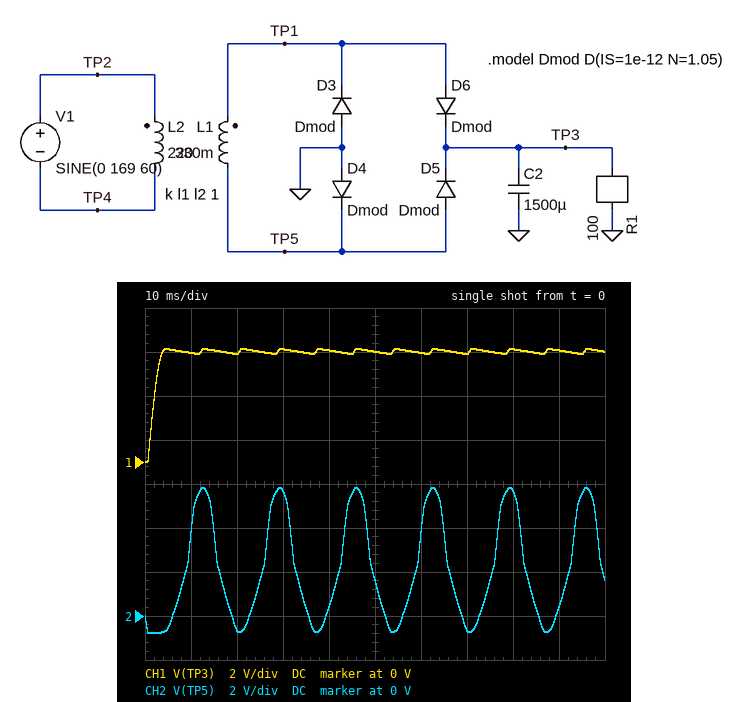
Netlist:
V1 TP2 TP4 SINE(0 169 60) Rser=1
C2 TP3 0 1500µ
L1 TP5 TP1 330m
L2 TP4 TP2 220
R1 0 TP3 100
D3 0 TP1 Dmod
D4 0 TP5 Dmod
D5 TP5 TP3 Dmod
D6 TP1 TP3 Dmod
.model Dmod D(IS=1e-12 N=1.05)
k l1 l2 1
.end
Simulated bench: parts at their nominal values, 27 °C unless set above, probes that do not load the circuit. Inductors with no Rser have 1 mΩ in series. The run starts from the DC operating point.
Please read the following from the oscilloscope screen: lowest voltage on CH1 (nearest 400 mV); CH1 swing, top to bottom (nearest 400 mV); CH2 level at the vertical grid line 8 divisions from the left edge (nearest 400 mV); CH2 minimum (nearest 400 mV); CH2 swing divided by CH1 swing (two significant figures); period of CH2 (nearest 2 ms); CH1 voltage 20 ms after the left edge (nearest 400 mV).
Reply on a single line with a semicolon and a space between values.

0 V; 5.2 V; 5.6 V; -800 mV; 1.3; 16 ms; 4.8 V
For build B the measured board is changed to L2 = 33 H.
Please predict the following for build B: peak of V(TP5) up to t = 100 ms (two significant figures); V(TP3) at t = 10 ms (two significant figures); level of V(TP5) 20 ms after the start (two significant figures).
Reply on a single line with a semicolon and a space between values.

16 V; 15 V; -670 mV
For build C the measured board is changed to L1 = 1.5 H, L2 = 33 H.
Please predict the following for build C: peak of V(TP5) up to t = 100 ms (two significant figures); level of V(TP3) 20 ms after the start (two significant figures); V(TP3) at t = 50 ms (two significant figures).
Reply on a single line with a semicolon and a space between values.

35 V; 33 V; 34 V
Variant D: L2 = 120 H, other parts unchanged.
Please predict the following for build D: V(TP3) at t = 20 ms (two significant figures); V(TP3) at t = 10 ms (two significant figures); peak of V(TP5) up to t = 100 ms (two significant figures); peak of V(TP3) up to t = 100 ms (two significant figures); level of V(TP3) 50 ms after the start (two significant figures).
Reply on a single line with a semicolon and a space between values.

7.1 V; 7.2 V; 8.1 V; 7.4 V; 7.3 V
